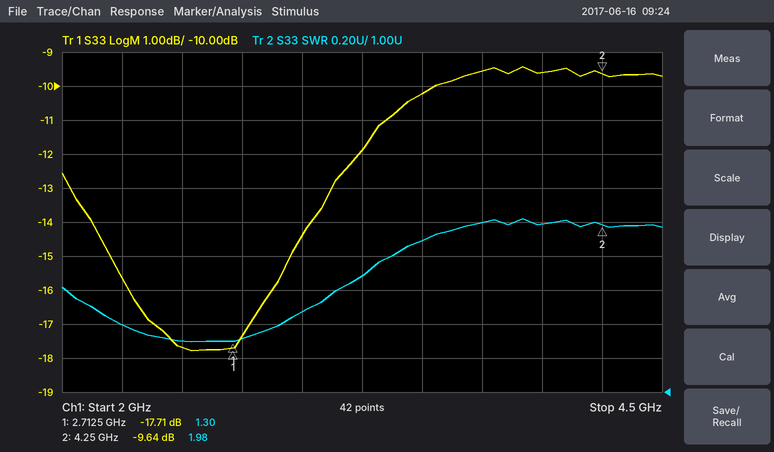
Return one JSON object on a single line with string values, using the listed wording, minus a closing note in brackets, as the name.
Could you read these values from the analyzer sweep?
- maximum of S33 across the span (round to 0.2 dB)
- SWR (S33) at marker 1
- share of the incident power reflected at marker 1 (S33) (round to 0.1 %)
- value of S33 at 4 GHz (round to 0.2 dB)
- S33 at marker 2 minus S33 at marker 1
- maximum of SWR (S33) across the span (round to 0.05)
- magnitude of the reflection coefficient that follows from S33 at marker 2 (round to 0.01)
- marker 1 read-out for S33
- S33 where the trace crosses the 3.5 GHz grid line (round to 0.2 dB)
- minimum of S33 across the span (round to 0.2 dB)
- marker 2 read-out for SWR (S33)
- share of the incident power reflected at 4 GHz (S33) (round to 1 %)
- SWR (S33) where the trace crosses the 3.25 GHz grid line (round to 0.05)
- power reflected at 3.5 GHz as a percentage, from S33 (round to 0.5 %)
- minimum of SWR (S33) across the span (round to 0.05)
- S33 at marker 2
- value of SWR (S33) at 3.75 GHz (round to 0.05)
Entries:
{"maximum of S33 across the span": "-9.4 dB", "SWR (S33) at marker 1": "1.30", "share of the incident power reflected at marker 1 (S33)": "1.7 %", "value of S33 at 4 GHz": "-9.6 dB", "S33 at marker 2 minus S33 at marker 1": "8.07 dB", "maximum of SWR (S33) across the span": "2.00", "magnitude of the reflection coefficient that follows from S33 at marker 2": "0.33", "marker 1 read-out for S33": "-17.71 dB", "S33 where the trace crosses the 3.5 GHz grid line": "-10.2 dB", "minimum of S33 across the span": "-17.8 dB", "marker 2 read-out for SWR": "1.98", "share of the incident power reflected at 4 GHz (S33)": "11 %", "SWR (S33) where the trace crosses the 3.25 GHz grid line": "1.70", "power reflected at 3.5 GHz as a percentage, from S33": "9.5 %", "minimum of SWR (S33) across the span": "1.30", "S33 at marker 2": "-9.64 dB", "value of SWR (S33) at 3.75 GHz": "2.00"}
